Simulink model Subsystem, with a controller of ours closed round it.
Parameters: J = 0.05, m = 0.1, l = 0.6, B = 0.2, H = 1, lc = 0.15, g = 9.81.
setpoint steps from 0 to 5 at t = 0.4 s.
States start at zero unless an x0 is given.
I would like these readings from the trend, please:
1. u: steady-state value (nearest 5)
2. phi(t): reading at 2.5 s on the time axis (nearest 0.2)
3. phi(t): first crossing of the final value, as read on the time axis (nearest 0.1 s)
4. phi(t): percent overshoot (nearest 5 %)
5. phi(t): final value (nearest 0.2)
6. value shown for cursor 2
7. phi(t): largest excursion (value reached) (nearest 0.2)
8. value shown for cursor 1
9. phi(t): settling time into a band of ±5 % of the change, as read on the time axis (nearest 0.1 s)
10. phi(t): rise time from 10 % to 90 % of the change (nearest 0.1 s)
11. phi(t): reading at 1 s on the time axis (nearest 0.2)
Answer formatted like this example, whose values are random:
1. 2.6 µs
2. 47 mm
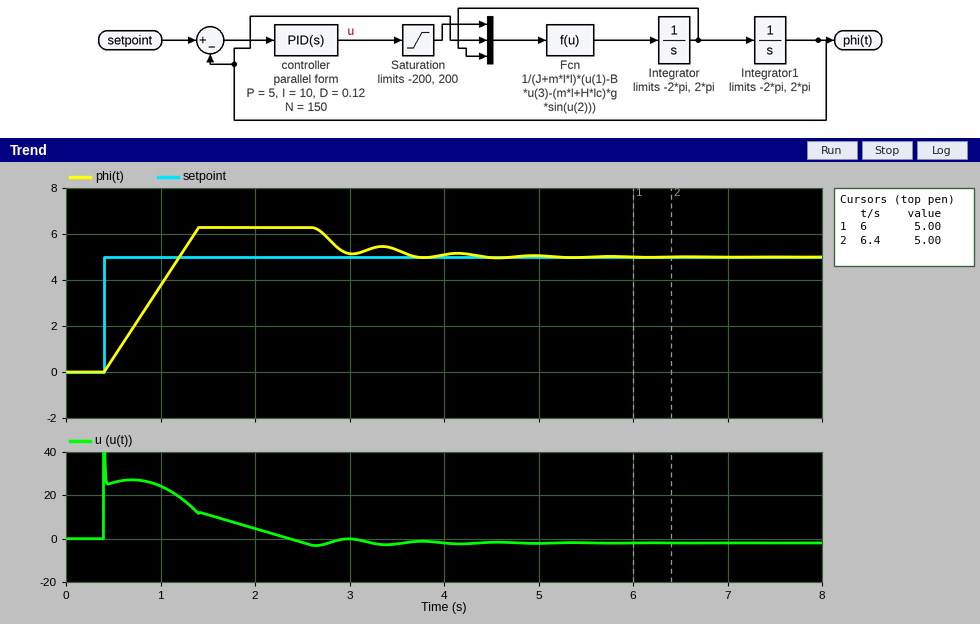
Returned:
1. 0
2. 6.2
3. 1.2 s
4. 25 %
5. 5.0
6. 5.00
7. 6.2
8. 5.00
9. 3.5 s
10. 0.6 s
11. 3.8
